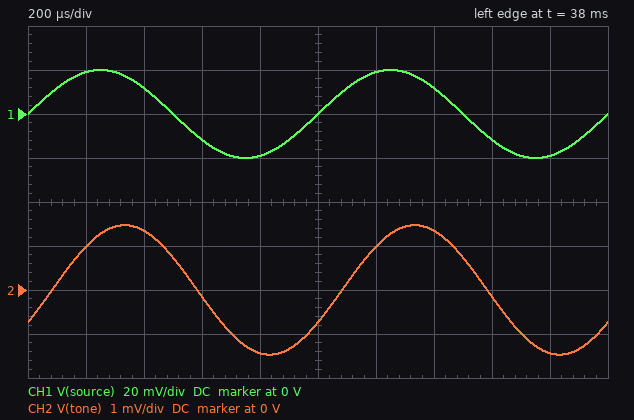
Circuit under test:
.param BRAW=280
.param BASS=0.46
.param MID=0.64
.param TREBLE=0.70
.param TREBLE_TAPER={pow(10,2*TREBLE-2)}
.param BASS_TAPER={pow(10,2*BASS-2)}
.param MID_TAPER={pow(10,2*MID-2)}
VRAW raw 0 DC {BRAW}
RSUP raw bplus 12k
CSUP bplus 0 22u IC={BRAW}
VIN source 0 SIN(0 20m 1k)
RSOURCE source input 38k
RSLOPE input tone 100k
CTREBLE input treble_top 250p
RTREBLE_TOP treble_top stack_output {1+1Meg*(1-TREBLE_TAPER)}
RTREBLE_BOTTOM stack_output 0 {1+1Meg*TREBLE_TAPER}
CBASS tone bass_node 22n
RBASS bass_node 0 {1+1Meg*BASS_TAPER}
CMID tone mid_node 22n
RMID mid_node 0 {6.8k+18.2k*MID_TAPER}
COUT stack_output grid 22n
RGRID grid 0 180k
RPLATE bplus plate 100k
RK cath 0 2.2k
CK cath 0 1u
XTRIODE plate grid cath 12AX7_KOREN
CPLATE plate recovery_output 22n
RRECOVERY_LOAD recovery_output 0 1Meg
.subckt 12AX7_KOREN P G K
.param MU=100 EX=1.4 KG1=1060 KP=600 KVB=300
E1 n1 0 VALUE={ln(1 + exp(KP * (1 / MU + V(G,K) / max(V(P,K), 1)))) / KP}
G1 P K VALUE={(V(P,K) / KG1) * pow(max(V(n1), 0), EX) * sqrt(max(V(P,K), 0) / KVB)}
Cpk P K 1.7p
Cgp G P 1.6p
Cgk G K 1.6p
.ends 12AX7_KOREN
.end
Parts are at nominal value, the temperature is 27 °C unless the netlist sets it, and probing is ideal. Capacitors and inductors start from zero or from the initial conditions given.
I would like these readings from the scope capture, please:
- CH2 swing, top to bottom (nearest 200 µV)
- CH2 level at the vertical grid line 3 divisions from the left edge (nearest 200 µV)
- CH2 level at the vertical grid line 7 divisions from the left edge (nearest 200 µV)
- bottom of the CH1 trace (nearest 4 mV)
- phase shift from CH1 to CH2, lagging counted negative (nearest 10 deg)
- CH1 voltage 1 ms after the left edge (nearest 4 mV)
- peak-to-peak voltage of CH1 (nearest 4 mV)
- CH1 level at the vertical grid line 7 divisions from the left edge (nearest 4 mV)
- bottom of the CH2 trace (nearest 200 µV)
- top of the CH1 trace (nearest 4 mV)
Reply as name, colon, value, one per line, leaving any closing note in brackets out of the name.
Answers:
CH2 swing, top to bottom: 3.0 mV
CH2 level at the vertical grid line 3 divisions from the left edge: -200 µV
CH2 level at the vertical grid line 7 divisions from the left edge: 1.4 mV
bottom of the CH1 trace: -20 mV
phase shift from CH1 to CH2, lagging counted negative: -30 deg
CH1 voltage 1 ms after the left edge: 0 V
peak-to-peak voltage of CH1: 40 mV
CH1 level at the vertical grid line 7 divisions from the left edge: 12 mV
bottom of the CH2 trace: -1.4 mV
top of the CH1 trace: 20 mV
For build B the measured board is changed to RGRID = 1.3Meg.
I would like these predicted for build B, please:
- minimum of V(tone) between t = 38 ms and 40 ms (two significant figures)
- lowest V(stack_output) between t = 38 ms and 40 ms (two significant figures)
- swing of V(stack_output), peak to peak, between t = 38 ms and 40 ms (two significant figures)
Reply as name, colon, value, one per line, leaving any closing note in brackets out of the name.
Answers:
minimum of V(tone) between t = 38 ms and 40 ms: -1.5 mV
lowest V(stack_output) between t = 38 ms and 40 ms: -3.4 mV
swing of V(stack_output), peak to peak, between t = 38 ms and 40 ms: 5.3 mV
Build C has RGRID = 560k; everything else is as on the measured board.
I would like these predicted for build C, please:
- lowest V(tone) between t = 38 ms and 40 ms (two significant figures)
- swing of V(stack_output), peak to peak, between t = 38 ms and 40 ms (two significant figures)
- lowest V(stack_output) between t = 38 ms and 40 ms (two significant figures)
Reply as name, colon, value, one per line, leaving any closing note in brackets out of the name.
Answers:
lowest V(tone) between t = 38 ms and 40 ms: -1.5 mV
swing of V(stack_output), peak to peak, between t = 38 ms and 40 ms: 4.5 mV
lowest V(stack_output) between t = 38 ms and 40 ms: -2.7 mV
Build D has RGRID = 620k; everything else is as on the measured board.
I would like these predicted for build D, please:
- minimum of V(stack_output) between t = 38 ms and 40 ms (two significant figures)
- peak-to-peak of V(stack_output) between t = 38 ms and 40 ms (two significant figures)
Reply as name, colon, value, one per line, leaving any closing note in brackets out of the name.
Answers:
minimum of V(stack_output) between t = 38 ms and 40 ms: -2.8 mV
peak-to-peak of V(stack_output) between t = 38 ms and 40 ms: 4.6 mV
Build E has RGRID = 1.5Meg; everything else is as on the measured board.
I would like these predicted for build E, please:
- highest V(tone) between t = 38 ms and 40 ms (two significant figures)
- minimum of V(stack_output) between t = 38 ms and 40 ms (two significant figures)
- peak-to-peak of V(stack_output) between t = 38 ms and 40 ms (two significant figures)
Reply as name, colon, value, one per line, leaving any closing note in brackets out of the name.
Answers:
highest V(tone) between t = 38 ms and 40 ms: 1.5 mV
minimum of V(stack_output) between t = 38 ms and 40 ms: -3.5 mV
peak-to-peak of V(stack_output) between t = 38 ms and 40 ms: 5.4 mV
